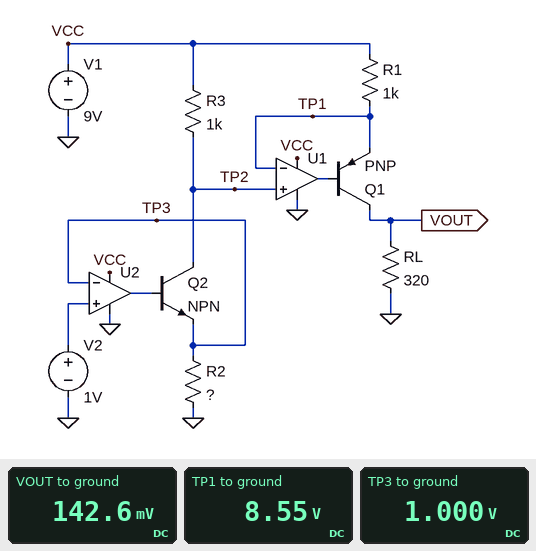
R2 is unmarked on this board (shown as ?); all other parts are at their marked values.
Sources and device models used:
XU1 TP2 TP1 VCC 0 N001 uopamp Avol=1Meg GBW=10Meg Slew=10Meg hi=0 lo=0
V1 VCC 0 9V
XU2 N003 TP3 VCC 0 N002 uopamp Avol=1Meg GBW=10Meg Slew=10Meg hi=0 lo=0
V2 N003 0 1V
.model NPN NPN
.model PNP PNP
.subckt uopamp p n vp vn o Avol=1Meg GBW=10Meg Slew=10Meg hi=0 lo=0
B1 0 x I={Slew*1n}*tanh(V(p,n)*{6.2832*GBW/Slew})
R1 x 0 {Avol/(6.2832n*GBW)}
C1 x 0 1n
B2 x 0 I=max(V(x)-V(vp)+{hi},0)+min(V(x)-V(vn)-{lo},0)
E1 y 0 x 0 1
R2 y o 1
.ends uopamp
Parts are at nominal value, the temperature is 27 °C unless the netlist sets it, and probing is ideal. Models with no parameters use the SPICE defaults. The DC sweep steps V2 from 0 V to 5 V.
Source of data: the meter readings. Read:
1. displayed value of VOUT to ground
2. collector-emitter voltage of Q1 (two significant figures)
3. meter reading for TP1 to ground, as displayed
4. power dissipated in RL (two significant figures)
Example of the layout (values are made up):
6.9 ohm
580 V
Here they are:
142.6 mV
-8.4 V
8.55 V
64 µW
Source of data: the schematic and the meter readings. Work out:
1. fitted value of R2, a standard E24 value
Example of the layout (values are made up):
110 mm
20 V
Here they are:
2.2 kΩ
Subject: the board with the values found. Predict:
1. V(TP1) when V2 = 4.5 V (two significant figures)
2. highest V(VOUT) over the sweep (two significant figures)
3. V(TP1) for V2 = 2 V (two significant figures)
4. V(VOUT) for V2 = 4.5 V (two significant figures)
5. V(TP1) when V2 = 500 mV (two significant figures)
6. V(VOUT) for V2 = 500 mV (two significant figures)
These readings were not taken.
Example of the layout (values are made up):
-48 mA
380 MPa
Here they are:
7.0 V
710 mV
8.1 V
640 mV
8.8 V
71 mV
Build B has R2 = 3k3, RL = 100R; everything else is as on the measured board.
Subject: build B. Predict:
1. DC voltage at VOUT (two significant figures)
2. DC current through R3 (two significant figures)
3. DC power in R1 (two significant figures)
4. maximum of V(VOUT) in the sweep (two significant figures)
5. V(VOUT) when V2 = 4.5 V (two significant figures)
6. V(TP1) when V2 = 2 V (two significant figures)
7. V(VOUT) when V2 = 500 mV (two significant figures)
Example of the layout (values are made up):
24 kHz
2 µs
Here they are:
30 mV
300 µA
90 µW
150 mV
130 mV
8.4 V
15 mV
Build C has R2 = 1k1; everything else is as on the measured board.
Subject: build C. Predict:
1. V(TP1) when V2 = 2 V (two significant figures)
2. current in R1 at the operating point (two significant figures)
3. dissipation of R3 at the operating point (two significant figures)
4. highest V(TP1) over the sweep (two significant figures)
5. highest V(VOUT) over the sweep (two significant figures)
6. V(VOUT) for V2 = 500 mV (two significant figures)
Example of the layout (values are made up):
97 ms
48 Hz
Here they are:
7.2 V
900 µA
810 µW
9.0 V
1.3 V
140 mV
